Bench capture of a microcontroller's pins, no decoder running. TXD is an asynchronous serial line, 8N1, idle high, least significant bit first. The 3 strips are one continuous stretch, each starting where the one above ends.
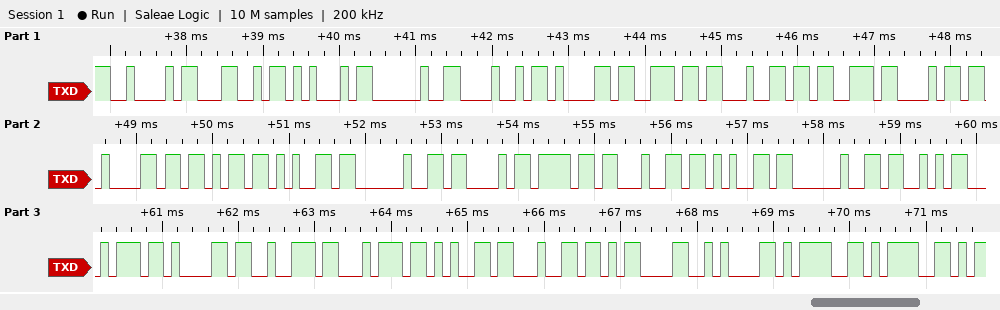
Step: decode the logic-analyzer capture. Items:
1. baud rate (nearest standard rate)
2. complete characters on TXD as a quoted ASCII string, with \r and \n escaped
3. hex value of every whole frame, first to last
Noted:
9600 baud
"BLE Handshake Code Started\r\n=="
0x42 0x4C 0x45 0x20 0x48 0x61 0x6E 0x64 0x73 0x68 0x61 0x6B 0x65 0x20 0x43 0x6F 0x64 0x65 0x20 0x53 0x74 0x61 0x72 0x74 0x65 0x64 0x0D 0x0A 0x3D 0x3D
